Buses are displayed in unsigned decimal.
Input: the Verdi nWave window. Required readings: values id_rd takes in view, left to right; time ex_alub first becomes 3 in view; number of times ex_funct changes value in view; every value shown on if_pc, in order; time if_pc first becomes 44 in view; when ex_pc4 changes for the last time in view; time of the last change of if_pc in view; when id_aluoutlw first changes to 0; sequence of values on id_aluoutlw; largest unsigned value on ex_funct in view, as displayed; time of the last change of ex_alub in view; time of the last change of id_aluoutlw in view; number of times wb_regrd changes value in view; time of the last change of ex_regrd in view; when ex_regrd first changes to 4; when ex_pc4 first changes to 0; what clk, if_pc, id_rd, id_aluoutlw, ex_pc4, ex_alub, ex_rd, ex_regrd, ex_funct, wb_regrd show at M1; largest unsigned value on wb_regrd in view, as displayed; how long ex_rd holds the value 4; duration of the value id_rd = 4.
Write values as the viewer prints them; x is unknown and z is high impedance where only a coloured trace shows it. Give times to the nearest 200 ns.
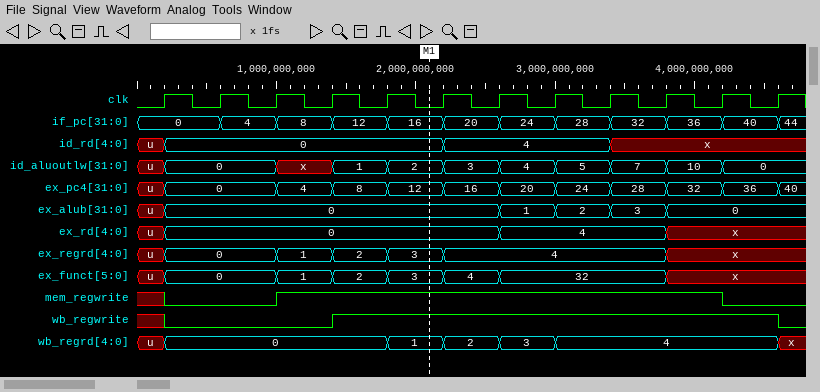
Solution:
u, 0, 4, x
3400 ns
7
0, 4, 8, 12, 16, 20, 24, 28, 32, 36, 40, 44
4600 ns
4600 ns
4600 ns
200 ns
u, 0, x, 1, 2, 3, 4, 5, 7, 10, 0
32
3800 ns
4200 ns
6
3800 ns
2200 ns
200 ns
clk=0, if_pc=16, id_rd=0, id_aluoutlw=2, ex_pc4=12, ex_alub=0, ex_rd=0, ex_regrd=3, ex_funct=3, wb_regrd=1
4
1200 ns
1200 ns
